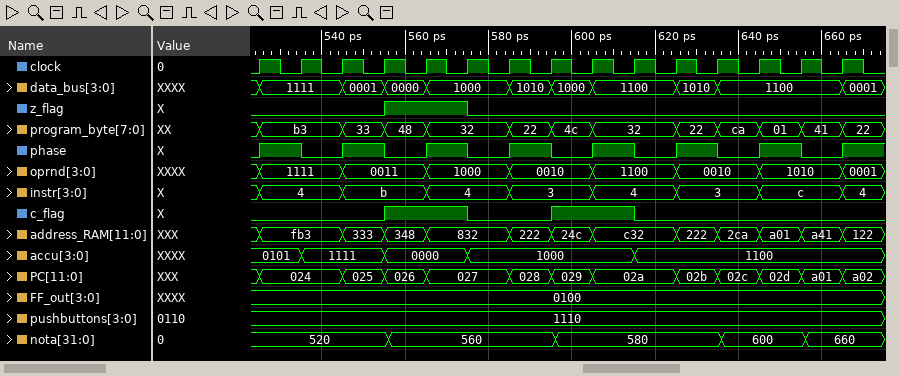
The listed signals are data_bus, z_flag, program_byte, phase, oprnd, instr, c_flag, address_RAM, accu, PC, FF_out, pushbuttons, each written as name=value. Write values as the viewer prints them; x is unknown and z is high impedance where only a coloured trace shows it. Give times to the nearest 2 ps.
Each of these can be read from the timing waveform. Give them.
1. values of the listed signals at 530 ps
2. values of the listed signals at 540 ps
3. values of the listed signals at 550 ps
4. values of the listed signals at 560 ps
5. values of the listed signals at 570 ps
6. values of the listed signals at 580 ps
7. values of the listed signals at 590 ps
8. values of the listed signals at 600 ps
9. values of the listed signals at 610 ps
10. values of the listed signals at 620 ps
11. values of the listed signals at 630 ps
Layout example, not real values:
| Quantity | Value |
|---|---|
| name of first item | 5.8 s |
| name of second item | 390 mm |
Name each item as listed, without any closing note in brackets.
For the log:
| Quantity | Value |
|---|---|
| values of the listed signals at 530 ps | data_bus=1111, z_flag=0, program_byte=b3, phase=1, oprnd=1111, instr=4, c_flag=0, address_RAM=fb3, accu=0101, PC=024, FF_out=0100, pushbuttons=1110 |
| values of the listed signals at 540 ps | data_bus=1111, z_flag=0, program_byte=b3, phase=0, oprnd=1111, instr=4, c_flag=0, address_RAM=fb3, accu=1111, PC=024, FF_out=0100, pushbuttons=1110 |
| values of the listed signals at 550 ps | data_bus=0001, z_flag=0, program_byte=33, phase=1, oprnd=0011, instr=b, c_flag=0, address_RAM=333, accu=1111, PC=025, FF_out=0100, pushbuttons=1110 |
| values of the listed signals at 560 ps | data_bus=0000, z_flag=1, program_byte=48, phase=0, oprnd=0011, instr=b, c_flag=1, address_RAM=348, accu=0000, PC=026, FF_out=0100, pushbuttons=1110 |
| values of the listed signals at 570 ps | data_bus=1000, z_flag=1, program_byte=32, phase=1, oprnd=1000, instr=4, c_flag=1, address_RAM=832, accu=0000, PC=027, FF_out=0100, pushbuttons=1110 |
| values of the listed signals at 580 ps | data_bus=1000, z_flag=0, program_byte=32, phase=0, oprnd=1000, instr=4, c_flag=0, address_RAM=832, accu=1000, PC=027, FF_out=0100, pushbuttons=1110 |
| values of the listed signals at 590 ps | data_bus=1010, z_flag=0, program_byte=22, phase=1, oprnd=0010, instr=3, c_flag=0, address_RAM=222, accu=1000, PC=028, FF_out=0100, pushbuttons=1110 |
| values of the listed signals at 600 ps | data_bus=1000, z_flag=0, program_byte=4c, phase=0, oprnd=0010, instr=3, c_flag=1, address_RAM=24c, accu=1000, PC=029, FF_out=0100, pushbuttons=1110 |
| values of the listed signals at 610 ps | data_bus=1100, z_flag=0, program_byte=32, phase=1, oprnd=1100, instr=4, c_flag=1, address_RAM=c32, accu=1000, PC=02a, FF_out=0100, pushbuttons=1110 |
| values of the listed signals at 620 ps | data_bus=1100, z_flag=0, program_byte=32, phase=0, oprnd=1100, instr=4, c_flag=0, address_RAM=c32, accu=1100, PC=02a, FF_out=0100, pushbuttons=1110 |
| values of the listed signals at 630 ps | data_bus=1010, z_flag=0, program_byte=22, phase=1, oprnd=0010, instr=3, c_flag=0, address_RAM=222, accu=1100, PC=02b, FF_out=0100, pushbuttons=1110 |
